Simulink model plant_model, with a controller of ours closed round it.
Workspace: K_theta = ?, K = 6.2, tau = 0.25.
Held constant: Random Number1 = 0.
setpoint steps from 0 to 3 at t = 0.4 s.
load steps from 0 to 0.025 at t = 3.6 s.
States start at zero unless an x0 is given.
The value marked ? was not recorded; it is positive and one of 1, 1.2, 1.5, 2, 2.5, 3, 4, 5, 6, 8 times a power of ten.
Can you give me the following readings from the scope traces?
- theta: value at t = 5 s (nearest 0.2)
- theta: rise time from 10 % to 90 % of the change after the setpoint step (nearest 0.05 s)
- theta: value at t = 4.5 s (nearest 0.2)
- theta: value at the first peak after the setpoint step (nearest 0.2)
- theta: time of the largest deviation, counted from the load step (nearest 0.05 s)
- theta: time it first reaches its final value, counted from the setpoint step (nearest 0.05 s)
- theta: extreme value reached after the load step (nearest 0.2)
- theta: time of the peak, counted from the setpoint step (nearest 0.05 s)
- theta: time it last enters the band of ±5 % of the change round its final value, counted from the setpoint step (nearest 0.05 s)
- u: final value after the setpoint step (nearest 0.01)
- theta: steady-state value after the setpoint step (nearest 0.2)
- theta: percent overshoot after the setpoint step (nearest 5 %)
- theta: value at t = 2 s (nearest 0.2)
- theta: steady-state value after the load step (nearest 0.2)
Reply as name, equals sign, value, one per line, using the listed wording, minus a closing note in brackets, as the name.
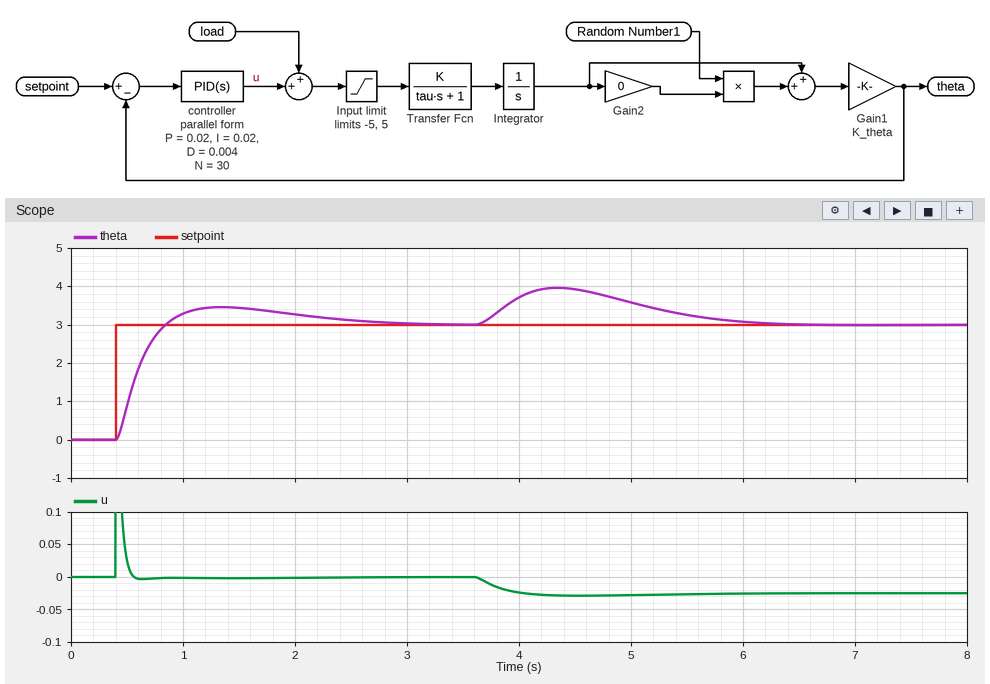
theta: value at t = 5 s = 3.6
theta: rise time from 10 % to 90 % of the change after the setpoint step = 0.30 s
theta: value at t = 4.5 s = 4.0
theta: value at the first peak after the setpoint step = 3.4
theta: time of the largest deviation, counted from the load step = 0.75 s
theta: time it first reaches its final value, counted from the setpoint step = 0.45 s
theta: extreme value reached after the load step = 4.0
theta: time of the peak, counted from the setpoint step = 0.95 s
theta: time it last enters the band of ±5 % of the change round its final value, counted from the setpoint step = 1.95 s
u: final value after the setpoint step = 0.00
theta: steady-state value after the setpoint step = 3.0
theta: percent overshoot after the setpoint step = 15 %
theta: value at t = 2 s = 3.2
theta: steady-state value after the load step = 3.0
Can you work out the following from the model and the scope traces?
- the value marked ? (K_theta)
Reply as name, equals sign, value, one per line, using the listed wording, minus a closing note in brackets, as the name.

the value marked ? = 40
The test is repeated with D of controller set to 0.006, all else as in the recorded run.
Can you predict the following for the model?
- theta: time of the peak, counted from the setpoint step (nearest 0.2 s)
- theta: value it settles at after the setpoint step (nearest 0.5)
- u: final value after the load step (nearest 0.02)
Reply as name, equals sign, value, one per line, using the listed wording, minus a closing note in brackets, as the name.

theta: time of the peak, counted from the setpoint step = 1.2 s
theta: value it settles at after the setpoint step = 3.0
u: final value after the load step = -0.02
